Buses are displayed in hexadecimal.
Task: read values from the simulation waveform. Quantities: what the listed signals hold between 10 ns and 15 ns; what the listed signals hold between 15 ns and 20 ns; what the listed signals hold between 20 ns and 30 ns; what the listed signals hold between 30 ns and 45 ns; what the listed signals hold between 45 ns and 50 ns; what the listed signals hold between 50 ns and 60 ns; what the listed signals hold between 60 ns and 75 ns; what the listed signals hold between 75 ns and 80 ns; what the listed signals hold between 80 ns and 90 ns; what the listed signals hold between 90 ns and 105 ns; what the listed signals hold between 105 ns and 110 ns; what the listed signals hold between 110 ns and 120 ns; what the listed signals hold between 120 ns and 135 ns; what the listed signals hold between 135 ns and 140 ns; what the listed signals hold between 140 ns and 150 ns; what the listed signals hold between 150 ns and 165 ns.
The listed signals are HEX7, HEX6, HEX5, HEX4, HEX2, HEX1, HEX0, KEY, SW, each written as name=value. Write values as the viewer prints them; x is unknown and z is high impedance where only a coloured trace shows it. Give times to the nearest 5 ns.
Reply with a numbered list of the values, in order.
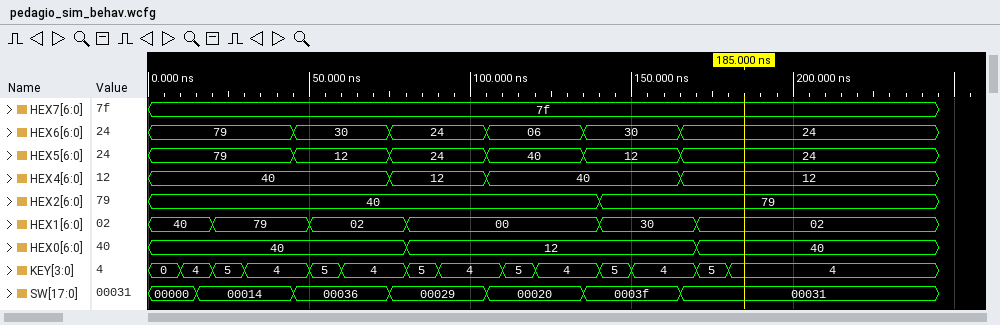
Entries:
1. HEX7=7f, HEX6=79, HEX5=79, HEX4=40, HEX2=40, HEX1=40, HEX0=40, KEY=4, SW=00000
2. HEX7=7f, HEX6=79, HEX5=79, HEX4=40, HEX2=40, HEX1=40, HEX0=40, KEY=4, SW=00014
3. HEX7=7f, HEX6=79, HEX5=79, HEX4=40, HEX2=40, HEX1=79, HEX0=40, KEY=5, SW=00014
4. HEX7=7f, HEX6=79, HEX5=79, HEX4=40, HEX2=40, HEX1=79, HEX0=40, KEY=4, SW=00014
5. HEX7=7f, HEX6=30, HEX5=12, HEX4=40, HEX2=40, HEX1=79, HEX0=40, KEY=4, SW=00036
6. HEX7=7f, HEX6=30, HEX5=12, HEX4=40, HEX2=40, HEX1=02, HEX0=40, KEY=5, SW=00036
7. HEX7=7f, HEX6=30, HEX5=12, HEX4=40, HEX2=40, HEX1=02, HEX0=40, KEY=4, SW=00036
8. HEX7=7f, HEX6=24, HEX5=24, HEX4=12, HEX2=40, HEX1=02, HEX0=40, KEY=4, SW=00029
9. HEX7=7f, HEX6=24, HEX5=24, HEX4=12, HEX2=40, HEX1=00, HEX0=12, KEY=5, SW=00029
10. HEX7=7f, HEX6=24, HEX5=24, HEX4=12, HEX2=40, HEX1=00, HEX0=12, KEY=4, SW=00029
11. HEX7=7f, HEX6=06, HEX5=40, HEX4=40, HEX2=40, HEX1=00, HEX0=12, KEY=4, SW=00020
12. HEX7=7f, HEX6=06, HEX5=40, HEX4=40, HEX2=40, HEX1=00, HEX0=12, KEY=5, SW=00020
13. HEX7=7f, HEX6=06, HEX5=40, HEX4=40, HEX2=40, HEX1=00, HEX0=12, KEY=4, SW=00020
14. HEX7=7f, HEX6=30, HEX5=12, HEX4=40, HEX2=40, HEX1=00, HEX0=12, KEY=4, SW=0003f
15. HEX7=7f, HEX6=30, HEX5=12, HEX4=40, HEX2=79, HEX1=30, HEX0=12, KEY=5, SW=0003f
16. HEX7=7f, HEX6=30, HEX5=12, HEX4=40, HEX2=79, HEX1=30, HEX0=12, KEY=4, SW=0003f
